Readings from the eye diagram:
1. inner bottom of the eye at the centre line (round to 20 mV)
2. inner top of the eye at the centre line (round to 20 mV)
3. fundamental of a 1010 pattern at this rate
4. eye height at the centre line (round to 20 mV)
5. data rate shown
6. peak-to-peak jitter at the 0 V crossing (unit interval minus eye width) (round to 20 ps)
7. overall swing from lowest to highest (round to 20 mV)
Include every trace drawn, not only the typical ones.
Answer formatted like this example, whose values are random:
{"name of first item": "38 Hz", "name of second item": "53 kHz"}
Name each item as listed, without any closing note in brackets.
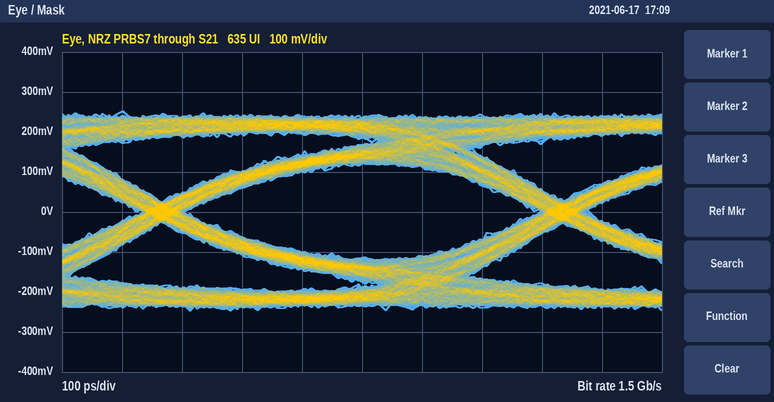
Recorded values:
{"inner bottom of the eye at the centre line": "-120 mV", "inner top of the eye at the centre line": "120 mV", "fundamental of a 1010 pattern at this rate": "750 MHz", "eye height at the centre line": "240 mV", "data rate shown": "1.5 Gb/s", "peak-to-peak jitter at the 0 V crossing (unit interval minus eye width)": "80 ps", "overall swing from lowest to highest": "500 mV"}
